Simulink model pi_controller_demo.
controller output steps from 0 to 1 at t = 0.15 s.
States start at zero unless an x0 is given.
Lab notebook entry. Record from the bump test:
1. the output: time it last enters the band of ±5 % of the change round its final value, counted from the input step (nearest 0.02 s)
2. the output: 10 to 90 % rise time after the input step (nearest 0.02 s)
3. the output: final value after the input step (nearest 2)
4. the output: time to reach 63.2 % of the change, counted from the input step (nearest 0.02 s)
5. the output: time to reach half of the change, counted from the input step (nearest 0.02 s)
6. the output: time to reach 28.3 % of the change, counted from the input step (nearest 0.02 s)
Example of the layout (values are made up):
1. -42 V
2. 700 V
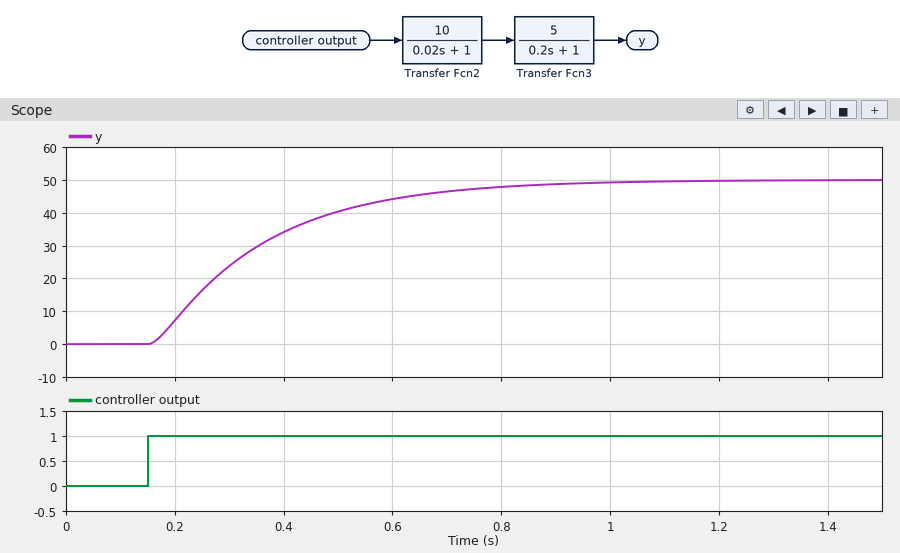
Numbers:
1. 0.62 s
2. 0.44 s
3. 50
4. 0.22 s
5. 0.16 s
6. 0.08 s
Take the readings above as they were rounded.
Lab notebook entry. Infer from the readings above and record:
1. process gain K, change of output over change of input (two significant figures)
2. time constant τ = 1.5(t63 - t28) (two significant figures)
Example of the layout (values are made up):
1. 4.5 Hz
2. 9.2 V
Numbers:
1. 50
2. 0.21 s
